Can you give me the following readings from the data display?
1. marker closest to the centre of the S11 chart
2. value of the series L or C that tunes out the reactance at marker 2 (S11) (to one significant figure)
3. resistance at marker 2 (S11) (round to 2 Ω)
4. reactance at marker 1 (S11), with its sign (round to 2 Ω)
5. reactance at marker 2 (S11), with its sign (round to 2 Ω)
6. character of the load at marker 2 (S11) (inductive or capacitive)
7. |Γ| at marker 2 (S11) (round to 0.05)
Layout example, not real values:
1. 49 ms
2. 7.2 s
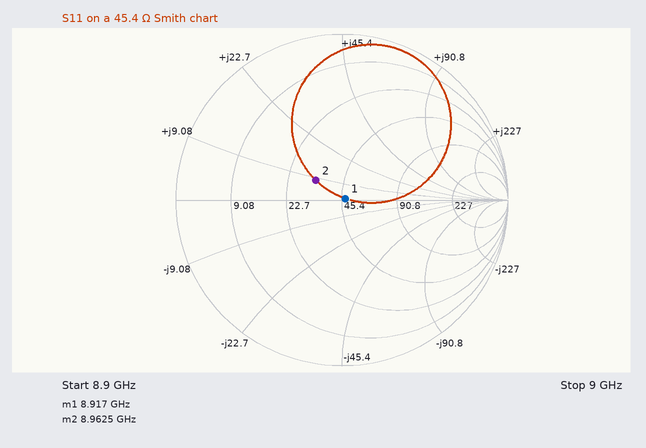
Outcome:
1. marker 1
2. 2 pF
3. 32 Ω
4. 0 Ω
5. +8 Ω
6. inductive
7. 0.20
